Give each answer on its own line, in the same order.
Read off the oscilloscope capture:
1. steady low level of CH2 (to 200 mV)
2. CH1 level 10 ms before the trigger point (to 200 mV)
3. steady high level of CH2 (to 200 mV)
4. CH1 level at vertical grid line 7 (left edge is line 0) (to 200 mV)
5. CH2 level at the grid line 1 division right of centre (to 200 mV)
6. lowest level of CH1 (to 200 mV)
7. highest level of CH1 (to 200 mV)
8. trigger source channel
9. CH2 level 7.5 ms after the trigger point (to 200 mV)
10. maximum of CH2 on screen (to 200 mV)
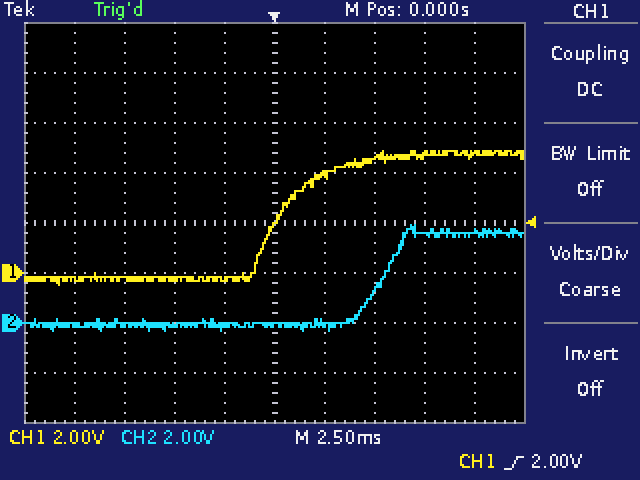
0.0 V
-200 mV
3.6 V
4.6 V
0.0 V
-400 mV
4.8 V
CH1
3.6 V
4.0 V
